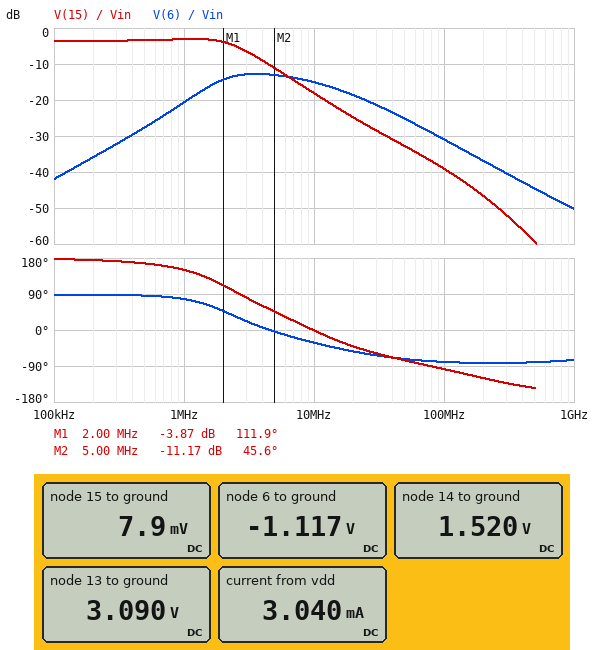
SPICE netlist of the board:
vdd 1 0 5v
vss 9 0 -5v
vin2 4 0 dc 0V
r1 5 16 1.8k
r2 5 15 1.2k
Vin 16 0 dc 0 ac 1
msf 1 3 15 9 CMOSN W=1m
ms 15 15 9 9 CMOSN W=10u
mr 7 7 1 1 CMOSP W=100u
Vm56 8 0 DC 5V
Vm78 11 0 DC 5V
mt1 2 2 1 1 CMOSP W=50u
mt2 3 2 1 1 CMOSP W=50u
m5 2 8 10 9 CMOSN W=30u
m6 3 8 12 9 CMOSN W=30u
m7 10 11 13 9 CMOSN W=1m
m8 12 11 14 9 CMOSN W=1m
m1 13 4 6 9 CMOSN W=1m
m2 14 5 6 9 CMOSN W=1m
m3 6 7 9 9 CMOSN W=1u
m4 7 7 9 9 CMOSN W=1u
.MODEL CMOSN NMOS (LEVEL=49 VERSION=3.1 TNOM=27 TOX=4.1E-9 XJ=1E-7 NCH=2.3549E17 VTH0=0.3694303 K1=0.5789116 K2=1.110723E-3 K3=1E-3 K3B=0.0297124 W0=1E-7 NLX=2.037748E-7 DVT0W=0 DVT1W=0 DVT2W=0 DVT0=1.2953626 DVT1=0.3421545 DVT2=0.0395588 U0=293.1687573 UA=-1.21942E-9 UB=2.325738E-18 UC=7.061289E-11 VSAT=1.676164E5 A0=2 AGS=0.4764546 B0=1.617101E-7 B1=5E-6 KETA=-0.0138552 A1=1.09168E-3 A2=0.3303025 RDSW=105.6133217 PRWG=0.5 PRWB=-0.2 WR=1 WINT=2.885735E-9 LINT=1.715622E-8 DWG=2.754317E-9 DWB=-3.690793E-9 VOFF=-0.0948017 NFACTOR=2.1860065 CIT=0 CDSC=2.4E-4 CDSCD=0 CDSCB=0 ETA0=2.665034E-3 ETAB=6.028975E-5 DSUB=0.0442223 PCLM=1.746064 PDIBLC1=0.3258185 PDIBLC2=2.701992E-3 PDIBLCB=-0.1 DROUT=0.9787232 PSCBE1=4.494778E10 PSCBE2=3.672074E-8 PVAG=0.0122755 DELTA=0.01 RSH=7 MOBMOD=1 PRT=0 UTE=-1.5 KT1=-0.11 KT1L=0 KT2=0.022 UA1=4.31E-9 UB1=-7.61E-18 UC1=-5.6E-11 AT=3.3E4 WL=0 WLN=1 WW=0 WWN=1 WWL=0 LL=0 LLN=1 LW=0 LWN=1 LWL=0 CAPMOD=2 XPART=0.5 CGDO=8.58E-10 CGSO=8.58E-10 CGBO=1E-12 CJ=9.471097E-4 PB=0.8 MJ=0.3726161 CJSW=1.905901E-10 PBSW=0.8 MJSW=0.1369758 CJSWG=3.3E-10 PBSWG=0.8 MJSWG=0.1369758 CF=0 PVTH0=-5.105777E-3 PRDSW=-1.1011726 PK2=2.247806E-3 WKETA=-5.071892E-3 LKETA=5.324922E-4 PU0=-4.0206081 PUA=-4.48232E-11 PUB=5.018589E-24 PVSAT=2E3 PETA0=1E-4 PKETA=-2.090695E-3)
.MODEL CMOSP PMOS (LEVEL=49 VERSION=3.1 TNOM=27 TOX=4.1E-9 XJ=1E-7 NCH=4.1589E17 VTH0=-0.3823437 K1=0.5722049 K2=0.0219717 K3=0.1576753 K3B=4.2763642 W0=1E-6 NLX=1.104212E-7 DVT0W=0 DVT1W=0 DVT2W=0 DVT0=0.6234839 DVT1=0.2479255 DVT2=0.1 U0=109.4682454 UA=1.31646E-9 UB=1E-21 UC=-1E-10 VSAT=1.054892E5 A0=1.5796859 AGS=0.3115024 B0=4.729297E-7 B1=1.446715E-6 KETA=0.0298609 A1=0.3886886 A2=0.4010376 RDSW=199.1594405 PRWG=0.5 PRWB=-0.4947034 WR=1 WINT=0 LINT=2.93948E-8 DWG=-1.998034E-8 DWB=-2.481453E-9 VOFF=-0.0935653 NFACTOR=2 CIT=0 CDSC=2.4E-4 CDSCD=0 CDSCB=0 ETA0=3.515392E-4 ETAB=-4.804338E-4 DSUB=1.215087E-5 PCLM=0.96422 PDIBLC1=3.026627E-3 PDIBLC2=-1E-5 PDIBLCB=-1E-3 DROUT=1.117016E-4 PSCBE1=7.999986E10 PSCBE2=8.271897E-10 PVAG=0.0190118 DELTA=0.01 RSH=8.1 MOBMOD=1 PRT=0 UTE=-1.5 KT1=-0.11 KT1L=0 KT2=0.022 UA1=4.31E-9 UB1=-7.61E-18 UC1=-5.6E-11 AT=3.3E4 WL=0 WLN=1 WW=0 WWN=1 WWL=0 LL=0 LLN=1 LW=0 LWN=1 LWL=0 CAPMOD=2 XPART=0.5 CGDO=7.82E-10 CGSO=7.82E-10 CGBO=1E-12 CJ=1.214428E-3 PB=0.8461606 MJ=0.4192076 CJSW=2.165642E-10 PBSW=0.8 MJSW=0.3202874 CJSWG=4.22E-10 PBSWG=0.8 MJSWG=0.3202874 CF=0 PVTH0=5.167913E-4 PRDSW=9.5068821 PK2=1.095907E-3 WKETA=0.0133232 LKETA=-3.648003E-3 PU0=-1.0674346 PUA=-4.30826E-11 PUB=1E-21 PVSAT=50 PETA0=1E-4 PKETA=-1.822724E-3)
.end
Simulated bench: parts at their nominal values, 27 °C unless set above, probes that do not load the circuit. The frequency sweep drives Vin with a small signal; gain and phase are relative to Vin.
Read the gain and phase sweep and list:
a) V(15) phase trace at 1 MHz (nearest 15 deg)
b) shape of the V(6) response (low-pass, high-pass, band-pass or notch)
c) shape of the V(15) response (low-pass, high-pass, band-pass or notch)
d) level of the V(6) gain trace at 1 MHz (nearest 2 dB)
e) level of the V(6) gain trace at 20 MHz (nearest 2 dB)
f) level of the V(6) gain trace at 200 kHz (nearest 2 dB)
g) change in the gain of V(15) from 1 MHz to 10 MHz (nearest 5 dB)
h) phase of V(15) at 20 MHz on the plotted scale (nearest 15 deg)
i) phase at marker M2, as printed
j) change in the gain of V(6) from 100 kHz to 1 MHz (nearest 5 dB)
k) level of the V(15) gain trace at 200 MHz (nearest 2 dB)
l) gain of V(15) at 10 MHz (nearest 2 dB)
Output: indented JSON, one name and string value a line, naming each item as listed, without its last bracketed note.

{
  "V(15) phase trace at 1 MHz": "150 deg",
  "shape of the V(6) response": "band-pass",
  "shape of the V(15) response": "low-pass",
  "level of the V(6) gain trace at 1 MHz": "-20 dB",
  "level of the V(6) gain trace at 20 MHz": "-18 dB",
  "level of the V(6) gain trace at 200 kHz": "-36 dB",
  "change in the gain of V(15) from 1 MHz to 10 MHz": "-15 dB",
  "phase of V(15) at 20 MHz on the plotted scale": "-45 deg",
  "phase at marker M2, as printed": "45.6 deg",
  "change in the gain of V(6) from 100 kHz to 1 MHz": "20 dB",
  "level of the V(15) gain trace at 200 MHz": "-46 dB",
  "gain of V(15) at 10 MHz": "-18 dB"
}
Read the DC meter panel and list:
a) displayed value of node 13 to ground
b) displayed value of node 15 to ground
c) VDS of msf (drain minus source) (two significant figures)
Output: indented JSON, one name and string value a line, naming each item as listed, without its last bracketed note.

{
  "displayed value of node 13 to ground": "3.090 V",
  "displayed value of node 15 to ground": "7.9 mV",
  "VDS of msf (drain minus source)": "5.0 V"
}
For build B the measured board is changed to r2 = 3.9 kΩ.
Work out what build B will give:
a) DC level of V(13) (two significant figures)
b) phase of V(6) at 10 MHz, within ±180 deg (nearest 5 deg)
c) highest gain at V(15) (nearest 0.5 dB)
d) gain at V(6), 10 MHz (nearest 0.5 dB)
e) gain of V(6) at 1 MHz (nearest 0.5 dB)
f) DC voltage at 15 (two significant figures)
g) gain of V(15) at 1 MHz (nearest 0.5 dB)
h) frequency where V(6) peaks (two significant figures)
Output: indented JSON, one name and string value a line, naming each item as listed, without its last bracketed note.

{
  "DC level of V(13)": "3.1 V",
  "phase of V(6) at 10 MHz, within ±180 deg": "-45 deg",
  "highest gain at V(15)": "6.5 dB",
  "gain at V(6), 10 MHz": "-13.5 dB",
  "gain of V(6) at 1 MHz": "-12.0 dB",
  "DC voltage at 15": "15 mV",
  "gain of V(15) at 1 MHz": "6.0 dB",
  "frequency where V(6) peaks": "2.2 MHz"
}
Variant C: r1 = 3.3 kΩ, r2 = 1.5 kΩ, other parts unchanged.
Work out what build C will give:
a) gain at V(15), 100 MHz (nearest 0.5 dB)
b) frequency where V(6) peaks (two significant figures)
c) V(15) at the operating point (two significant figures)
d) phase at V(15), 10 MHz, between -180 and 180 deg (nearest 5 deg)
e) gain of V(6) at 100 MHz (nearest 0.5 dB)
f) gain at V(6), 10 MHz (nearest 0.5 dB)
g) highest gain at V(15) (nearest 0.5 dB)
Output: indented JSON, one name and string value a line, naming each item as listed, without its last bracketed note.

{
  "gain at V(15), 100 MHz": "-46.0 dB",
  "frequency where V(6) peaks": "3.5 MHz",
  "V(15) at the operating point": "6.9 mV",
  "phase at V(15), 10 MHz, between -180 and 180 deg": "-10 deg",
  "gain of V(6) at 100 MHz": "-36.0 dB",
  "gain at V(6), 10 MHz": "-18.5 dB",
  "highest gain at V(15)": "-6.0 dB"
}
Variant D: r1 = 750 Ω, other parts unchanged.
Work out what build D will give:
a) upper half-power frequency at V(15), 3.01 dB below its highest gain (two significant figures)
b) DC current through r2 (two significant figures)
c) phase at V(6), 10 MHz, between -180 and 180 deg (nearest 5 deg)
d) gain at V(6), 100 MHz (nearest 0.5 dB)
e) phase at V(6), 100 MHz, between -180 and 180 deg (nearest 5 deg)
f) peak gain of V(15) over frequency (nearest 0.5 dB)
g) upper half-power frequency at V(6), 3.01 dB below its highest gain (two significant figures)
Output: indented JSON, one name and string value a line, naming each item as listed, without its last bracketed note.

{
  "upper half-power frequency at V(15), 3.01 dB below its highest gain": "1.8 MHz",
  "DC current through r2": "6.3 µA",
  "phase at V(6), 10 MHz, between -180 and 180 deg": "-20 deg",
  "gain at V(6), 100 MHz": "-23.5 dB",
  "phase at V(6), 100 MHz, between -180 and 180 deg": "-75 deg",
  "peak gain of V(15) over frequency": "4.0 dB",
  "upper half-power frequency at V(6), 3.01 dB below its highest gain": "19 MHz"
}
